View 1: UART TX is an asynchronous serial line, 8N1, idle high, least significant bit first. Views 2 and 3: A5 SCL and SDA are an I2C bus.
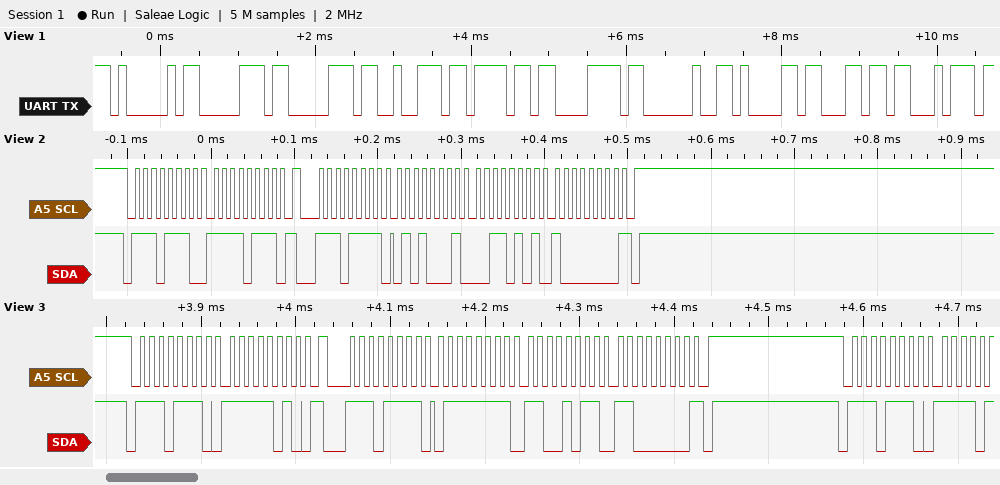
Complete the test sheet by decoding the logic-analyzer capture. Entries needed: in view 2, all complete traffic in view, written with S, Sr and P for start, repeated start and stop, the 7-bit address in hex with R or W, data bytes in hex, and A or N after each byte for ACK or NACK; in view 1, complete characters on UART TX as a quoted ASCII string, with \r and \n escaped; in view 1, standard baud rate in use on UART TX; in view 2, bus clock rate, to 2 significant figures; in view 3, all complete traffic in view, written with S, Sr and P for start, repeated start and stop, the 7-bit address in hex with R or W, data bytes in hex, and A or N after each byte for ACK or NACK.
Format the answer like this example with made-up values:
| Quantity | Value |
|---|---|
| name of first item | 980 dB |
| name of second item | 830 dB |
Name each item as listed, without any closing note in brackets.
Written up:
| Quantity | Value |
|---|---|
| in view 2, all complete traffic in view, written with S, Sr and P for start, repeated start and stop, the 7-bit address in hex with R or W, data bytes in hex, and A or N after each byte for ACK or NACK | S 77W A F7 A Sr 77R A 51 A 35 A 80 N P |
| in view 1, complete characters on UART TX as a quoted ASCII string, with \r and \n escaped | "Approx alt" |
| in view 1, standard baud rate in use on UART TX | 9600 baud |
| in view 2, bus clock rate, to 2 significant figures | 100 kHz |
| in view 3, all complete traffic in view, written with S, Sr and P for start, repeated start and stop, the 7-bit address in hex with R or W, data bytes in hex, and A or N after each byte for ACK or NACK | S 77W A FA A Sr 77R A 7F A CB A C0 N P S 77W A |
